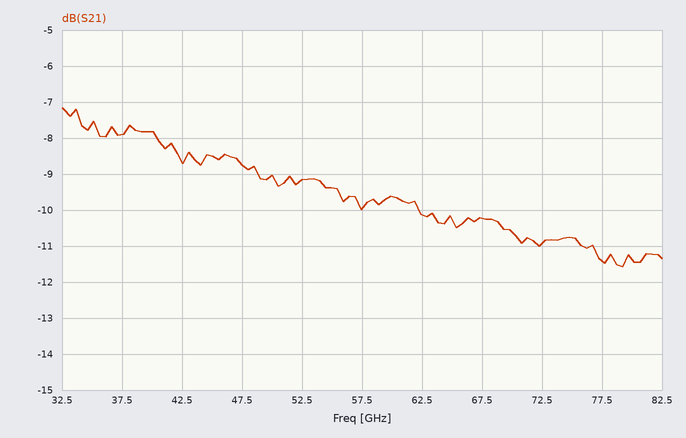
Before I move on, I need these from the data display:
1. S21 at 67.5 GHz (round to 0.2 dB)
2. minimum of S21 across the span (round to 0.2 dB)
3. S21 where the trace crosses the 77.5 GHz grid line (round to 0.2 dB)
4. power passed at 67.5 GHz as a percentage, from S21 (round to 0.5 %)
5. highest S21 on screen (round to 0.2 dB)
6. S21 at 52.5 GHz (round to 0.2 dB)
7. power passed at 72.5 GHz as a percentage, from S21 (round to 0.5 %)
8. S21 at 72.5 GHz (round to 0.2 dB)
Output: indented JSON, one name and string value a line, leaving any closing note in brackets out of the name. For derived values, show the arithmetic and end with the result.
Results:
{
  "S21 at 67.5 GHz": "-10.2 dB",
  "minimum of S21 across the span": "-11.6 dB",
  "S21 where the trace crosses the 77.5 GHz grid line": "-11.4 dB",
  "power passed at 67.5 GHz as a percentage, from S21": "10^(-10.2/10) ≈ 9.5 %",
  "highest S21 on screen": "-7.2 dB",
  "S21 at 52.5 GHz": "-9.2 dB",
  "power passed at 72.5 GHz as a percentage, from S21": "10^(-11/10) ≈ 7.94 %, so 8.0 % to the nearest 0.5 %",
  "S21 at 72.5 GHz": "-11.0 dB"
}
